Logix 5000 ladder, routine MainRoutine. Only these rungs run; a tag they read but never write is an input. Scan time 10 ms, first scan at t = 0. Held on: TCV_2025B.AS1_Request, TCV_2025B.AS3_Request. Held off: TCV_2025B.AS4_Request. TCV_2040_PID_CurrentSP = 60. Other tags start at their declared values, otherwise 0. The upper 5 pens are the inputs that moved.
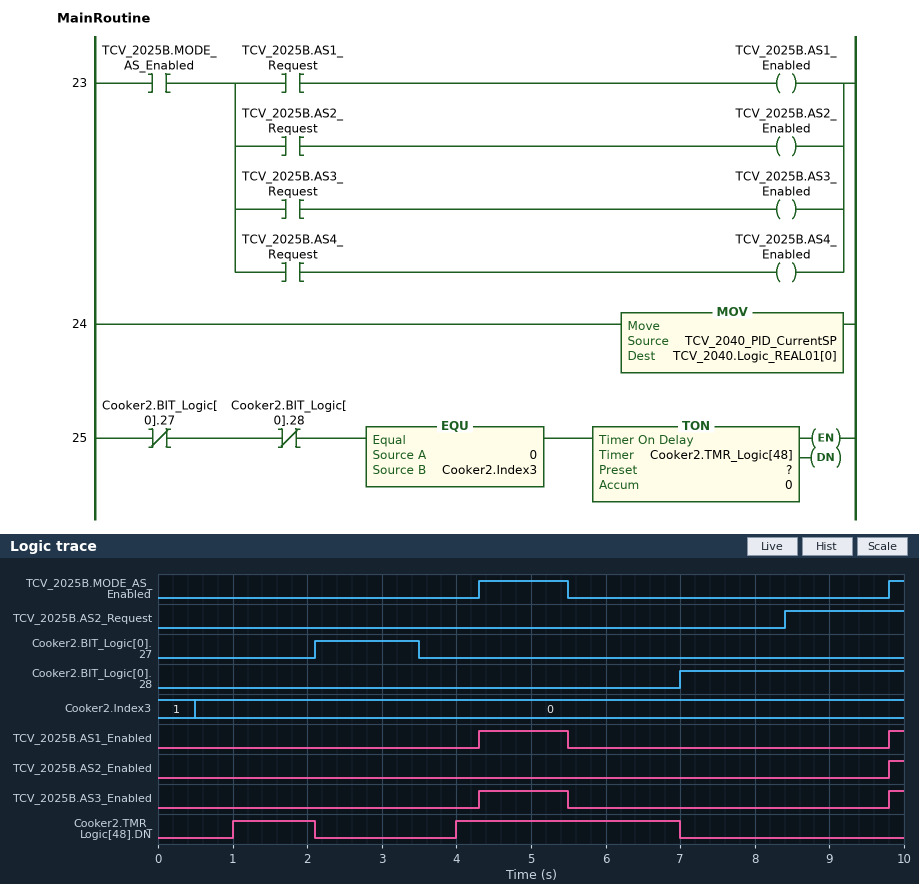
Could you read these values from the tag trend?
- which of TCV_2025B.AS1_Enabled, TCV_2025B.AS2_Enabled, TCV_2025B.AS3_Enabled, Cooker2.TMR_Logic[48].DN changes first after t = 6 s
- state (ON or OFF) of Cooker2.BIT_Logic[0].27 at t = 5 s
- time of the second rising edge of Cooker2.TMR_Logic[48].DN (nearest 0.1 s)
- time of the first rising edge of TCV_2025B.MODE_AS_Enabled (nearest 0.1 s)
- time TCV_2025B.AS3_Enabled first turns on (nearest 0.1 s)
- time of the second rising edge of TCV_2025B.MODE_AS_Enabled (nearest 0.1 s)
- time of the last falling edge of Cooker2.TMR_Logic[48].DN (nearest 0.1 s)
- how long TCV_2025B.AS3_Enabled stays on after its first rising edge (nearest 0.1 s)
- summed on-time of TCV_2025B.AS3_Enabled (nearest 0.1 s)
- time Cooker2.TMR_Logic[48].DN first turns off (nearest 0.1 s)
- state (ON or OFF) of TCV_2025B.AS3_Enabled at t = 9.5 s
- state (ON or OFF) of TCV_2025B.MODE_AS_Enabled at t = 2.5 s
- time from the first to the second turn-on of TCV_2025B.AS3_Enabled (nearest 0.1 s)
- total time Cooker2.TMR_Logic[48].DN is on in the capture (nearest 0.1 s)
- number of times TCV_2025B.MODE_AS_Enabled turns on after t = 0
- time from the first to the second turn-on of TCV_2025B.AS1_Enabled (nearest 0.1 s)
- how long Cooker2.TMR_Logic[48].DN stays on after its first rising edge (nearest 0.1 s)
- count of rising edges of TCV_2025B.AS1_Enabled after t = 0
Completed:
Cooker2.TMR_Logic[48].DN
OFF
4.0 s
4.3 s
4.3 s
9.8 s
7.0 s
1.2 s
1.4 s
2.1 s
OFF
OFF
5.5 s
4.1 s
2
5.5 s
1.1 s
2
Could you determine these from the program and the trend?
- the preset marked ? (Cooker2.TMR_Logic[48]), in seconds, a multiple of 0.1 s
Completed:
0.5 s
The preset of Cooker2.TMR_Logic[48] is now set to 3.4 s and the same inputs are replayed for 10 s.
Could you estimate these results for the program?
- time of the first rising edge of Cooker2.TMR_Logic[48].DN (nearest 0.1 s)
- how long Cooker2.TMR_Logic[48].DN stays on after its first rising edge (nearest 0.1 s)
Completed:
6.9 s
0.1 s
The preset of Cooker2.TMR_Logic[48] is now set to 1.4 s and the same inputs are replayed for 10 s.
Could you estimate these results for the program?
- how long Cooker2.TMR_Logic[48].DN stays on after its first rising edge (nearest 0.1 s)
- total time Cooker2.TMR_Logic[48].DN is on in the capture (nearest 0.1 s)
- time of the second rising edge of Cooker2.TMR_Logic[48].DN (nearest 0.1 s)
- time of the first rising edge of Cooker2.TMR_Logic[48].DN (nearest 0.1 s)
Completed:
0.2 s
2.3 s
4.9 s
1.9 s
